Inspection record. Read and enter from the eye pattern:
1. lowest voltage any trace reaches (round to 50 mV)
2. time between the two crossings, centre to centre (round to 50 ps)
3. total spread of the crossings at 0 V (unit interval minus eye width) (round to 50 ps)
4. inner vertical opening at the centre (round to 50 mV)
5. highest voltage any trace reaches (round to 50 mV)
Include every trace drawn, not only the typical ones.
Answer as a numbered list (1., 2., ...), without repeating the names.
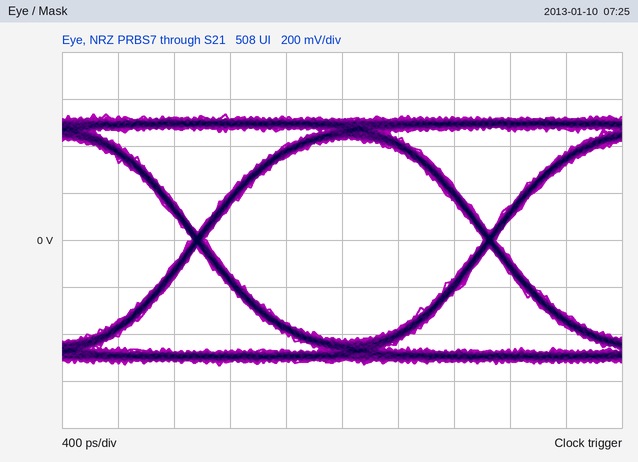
1. -550 mV
2. 2.10 ns
3. 100 ps
4. 850 mV
5. 550 mV
